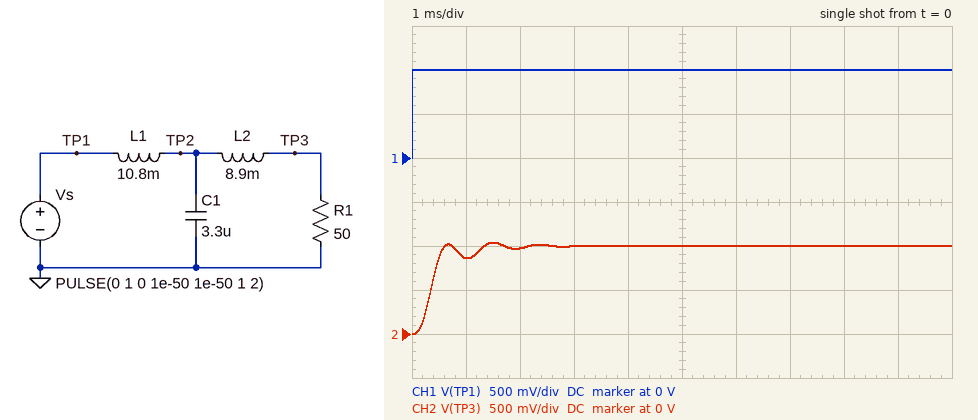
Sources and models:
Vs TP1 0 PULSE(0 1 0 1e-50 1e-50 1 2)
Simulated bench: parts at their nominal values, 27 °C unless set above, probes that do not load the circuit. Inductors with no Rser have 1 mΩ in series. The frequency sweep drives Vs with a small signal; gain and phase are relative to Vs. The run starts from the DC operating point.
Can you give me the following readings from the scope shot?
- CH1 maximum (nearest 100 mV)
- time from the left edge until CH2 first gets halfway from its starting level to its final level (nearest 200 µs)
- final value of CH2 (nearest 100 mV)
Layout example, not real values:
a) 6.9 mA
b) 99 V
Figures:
a) 1.0 V
b) 400 µs
c) 1.0 V
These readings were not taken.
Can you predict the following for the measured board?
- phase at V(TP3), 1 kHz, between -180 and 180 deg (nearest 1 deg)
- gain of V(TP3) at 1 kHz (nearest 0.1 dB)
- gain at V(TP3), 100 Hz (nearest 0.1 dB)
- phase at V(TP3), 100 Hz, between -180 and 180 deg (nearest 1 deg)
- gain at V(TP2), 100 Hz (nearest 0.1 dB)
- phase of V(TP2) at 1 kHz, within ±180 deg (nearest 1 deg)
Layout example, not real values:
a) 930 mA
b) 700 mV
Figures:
a) -114 deg
b) 0.1 dB
c) -0.1 dB
d) -14 deg
e) -0.1 dB
f) -66 deg
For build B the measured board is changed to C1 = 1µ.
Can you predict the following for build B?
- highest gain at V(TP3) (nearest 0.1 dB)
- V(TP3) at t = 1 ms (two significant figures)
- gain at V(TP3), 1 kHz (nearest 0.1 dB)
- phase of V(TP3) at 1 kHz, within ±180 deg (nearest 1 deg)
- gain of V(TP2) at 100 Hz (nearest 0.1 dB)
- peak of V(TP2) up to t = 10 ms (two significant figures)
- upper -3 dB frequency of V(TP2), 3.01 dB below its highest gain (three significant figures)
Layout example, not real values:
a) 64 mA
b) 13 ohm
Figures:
a) 0 dB
b) 890 mV
c) -6.4 dB
d) -74 deg
e) -0.2 dB
f) 1.1 V
g) 2.43 kHz
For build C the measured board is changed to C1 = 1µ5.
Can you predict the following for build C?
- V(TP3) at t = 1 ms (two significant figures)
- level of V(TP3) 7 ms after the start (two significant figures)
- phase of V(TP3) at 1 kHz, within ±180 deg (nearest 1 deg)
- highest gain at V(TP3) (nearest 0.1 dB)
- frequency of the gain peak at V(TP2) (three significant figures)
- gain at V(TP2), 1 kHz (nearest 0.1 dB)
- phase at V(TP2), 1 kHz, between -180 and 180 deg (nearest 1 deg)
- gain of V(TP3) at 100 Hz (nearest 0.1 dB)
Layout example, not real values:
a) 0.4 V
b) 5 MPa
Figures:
a) 990 mV
b) 1.0 V
c) -78 deg
d) 0 dB
e) 1.77 kHz
f) -1.6 dB
g) -30 deg
h) -0.2 dB
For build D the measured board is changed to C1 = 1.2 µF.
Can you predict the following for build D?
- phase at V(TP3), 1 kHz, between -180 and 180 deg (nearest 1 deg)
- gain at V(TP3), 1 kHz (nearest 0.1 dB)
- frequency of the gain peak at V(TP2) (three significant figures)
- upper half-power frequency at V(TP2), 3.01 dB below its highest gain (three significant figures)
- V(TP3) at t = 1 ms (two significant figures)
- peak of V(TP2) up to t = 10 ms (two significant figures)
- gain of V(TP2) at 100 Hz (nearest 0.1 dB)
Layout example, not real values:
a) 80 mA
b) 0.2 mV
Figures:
a) -76 deg
b) -5.9 dB
c) 2.00 kHz
d) 2.22 kHz
e) 930 mV
f) 1.1 V
g) -0.2 dB
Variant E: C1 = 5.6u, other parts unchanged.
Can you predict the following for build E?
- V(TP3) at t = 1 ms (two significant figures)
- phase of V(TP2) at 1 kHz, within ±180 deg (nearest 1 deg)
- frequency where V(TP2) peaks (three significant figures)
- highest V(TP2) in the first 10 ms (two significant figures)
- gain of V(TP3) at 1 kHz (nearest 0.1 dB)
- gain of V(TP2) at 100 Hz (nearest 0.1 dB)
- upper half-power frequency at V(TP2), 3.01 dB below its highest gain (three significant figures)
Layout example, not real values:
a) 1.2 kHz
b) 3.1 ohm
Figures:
a) 1.1 V
b) -140 deg
c) 798 Hz
d) 1.3 V
e) -2.9 dB
f) 0 dB
g) 973 Hz
